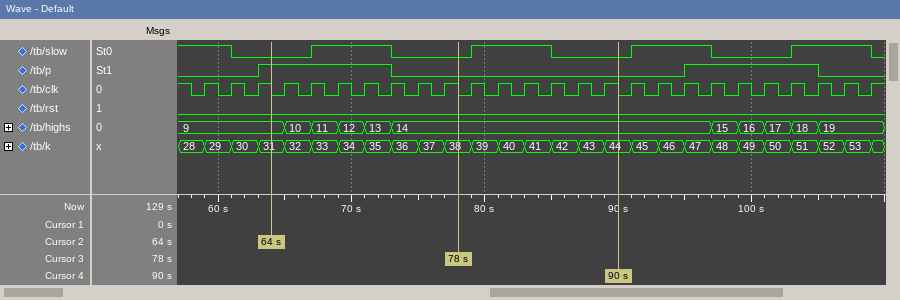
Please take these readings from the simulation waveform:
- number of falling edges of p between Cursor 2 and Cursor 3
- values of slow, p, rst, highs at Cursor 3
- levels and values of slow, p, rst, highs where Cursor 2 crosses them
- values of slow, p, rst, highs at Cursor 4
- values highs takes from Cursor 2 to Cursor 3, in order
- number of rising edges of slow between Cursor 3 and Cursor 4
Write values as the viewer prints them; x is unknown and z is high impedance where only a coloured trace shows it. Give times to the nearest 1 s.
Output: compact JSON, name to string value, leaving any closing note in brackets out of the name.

{"number of falling edges of p between Cursor 2 and Cursor 3": "1", "values of slow, p, rst, highs at Cursor 3": "slow=0, p=0, rst=0, highs=14", "levels and values of slow, p, rst, highs where Cursor 2 crosses them": "slow=0, p=1, rst=0, highs=9", "values of slow, p, rst, highs at Cursor 4": "slow=0, p=0, rst=0, highs=14", "values highs takes from Cursor 2 to Cursor 3, in order": "9, 10, 11, 12, 13, 14", "number of rising edges of slow between Cursor 3 and Cursor 4": "1"}
